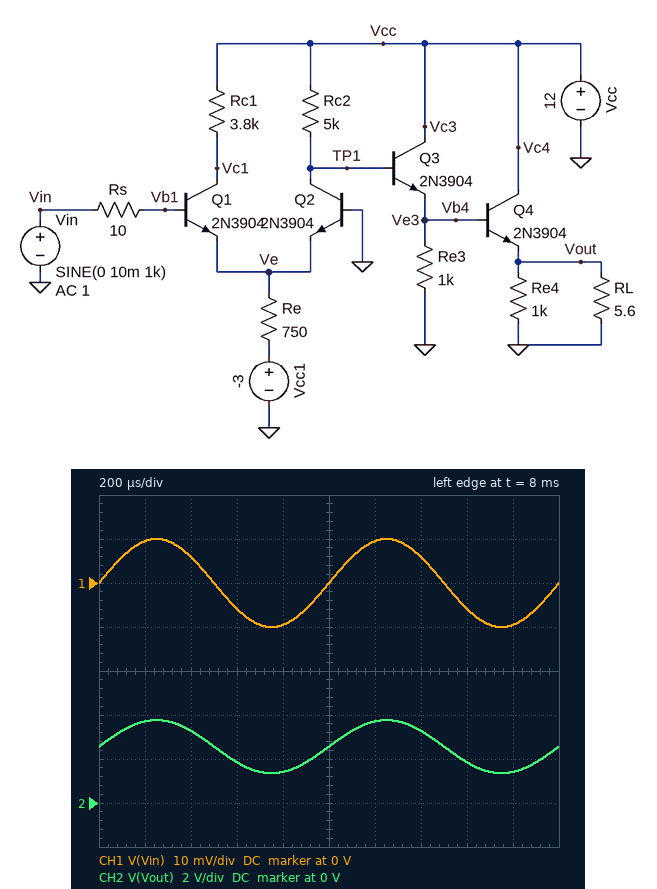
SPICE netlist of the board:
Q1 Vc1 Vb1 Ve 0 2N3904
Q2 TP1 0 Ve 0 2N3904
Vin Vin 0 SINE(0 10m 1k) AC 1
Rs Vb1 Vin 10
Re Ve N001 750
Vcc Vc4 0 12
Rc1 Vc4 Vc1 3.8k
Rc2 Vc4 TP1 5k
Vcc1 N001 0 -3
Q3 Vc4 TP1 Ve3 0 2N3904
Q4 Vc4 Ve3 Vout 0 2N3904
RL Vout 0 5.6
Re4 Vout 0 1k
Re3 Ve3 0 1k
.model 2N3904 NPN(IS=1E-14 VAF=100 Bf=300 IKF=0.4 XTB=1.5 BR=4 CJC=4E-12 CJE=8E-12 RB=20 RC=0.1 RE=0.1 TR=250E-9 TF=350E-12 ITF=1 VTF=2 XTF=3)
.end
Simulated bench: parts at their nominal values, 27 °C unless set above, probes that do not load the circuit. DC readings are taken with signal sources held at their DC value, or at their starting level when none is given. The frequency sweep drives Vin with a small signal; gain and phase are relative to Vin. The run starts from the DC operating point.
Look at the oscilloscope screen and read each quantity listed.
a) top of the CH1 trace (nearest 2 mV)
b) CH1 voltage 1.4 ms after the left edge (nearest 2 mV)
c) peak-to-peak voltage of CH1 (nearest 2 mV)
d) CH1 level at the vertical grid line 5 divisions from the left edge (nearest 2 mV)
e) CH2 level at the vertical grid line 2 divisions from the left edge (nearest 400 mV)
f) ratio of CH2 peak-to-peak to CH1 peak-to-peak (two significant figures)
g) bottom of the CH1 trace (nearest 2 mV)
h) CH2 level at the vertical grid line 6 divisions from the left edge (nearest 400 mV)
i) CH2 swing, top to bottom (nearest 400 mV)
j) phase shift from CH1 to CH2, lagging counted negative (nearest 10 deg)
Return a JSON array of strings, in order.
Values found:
["10 mV", "6 mV", "20 mV", "0 V", "3.2 V", "120", "-10 mV", "3.6 V", "2.4 V", "0 deg"]
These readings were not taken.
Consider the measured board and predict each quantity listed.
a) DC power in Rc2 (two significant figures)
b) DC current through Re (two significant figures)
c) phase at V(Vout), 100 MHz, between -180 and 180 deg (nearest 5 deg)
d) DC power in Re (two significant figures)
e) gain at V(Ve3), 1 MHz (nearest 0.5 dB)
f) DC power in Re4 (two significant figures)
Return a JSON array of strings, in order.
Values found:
["12 mW", "3.1 mA", "-160 deg", "7.3 mW", "42.0 dB", "6.6 mW"]
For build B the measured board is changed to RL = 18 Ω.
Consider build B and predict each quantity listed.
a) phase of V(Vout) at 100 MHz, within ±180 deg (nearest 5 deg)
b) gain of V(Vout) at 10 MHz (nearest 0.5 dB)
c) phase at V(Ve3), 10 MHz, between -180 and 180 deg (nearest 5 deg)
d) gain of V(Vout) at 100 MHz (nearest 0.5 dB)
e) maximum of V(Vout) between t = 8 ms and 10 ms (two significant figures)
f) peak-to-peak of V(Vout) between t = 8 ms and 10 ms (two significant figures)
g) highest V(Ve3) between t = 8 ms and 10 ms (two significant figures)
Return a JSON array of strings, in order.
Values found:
["-145 deg", "35.0 dB", "-80 deg", "7.0 dB", "4.0 V", "2.6 V", "4.9 V"]
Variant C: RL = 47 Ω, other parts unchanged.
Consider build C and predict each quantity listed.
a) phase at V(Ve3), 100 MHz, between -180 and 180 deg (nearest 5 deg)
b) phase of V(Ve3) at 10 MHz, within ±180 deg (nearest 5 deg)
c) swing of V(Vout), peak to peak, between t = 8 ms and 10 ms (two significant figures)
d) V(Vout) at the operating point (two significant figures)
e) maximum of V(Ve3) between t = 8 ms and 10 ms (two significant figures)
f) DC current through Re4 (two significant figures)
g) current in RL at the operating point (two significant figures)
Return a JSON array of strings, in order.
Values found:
["-125 deg", "-75 deg", "2.6 V", "2.8 V", "4.9 V", "2.8 mA", "59 mA"]
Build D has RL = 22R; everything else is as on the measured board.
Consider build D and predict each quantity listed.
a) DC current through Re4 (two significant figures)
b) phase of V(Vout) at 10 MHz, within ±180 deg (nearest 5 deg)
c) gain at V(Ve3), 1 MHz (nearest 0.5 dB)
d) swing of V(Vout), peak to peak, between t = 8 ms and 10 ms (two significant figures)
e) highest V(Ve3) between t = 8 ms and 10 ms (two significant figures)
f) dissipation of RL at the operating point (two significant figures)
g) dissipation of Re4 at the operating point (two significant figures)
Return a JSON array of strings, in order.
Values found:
["2.7 mA", "-80 deg", "42.5 dB", "2.6 V", "4.9 V", "340 mW", "7.5 mW"]
